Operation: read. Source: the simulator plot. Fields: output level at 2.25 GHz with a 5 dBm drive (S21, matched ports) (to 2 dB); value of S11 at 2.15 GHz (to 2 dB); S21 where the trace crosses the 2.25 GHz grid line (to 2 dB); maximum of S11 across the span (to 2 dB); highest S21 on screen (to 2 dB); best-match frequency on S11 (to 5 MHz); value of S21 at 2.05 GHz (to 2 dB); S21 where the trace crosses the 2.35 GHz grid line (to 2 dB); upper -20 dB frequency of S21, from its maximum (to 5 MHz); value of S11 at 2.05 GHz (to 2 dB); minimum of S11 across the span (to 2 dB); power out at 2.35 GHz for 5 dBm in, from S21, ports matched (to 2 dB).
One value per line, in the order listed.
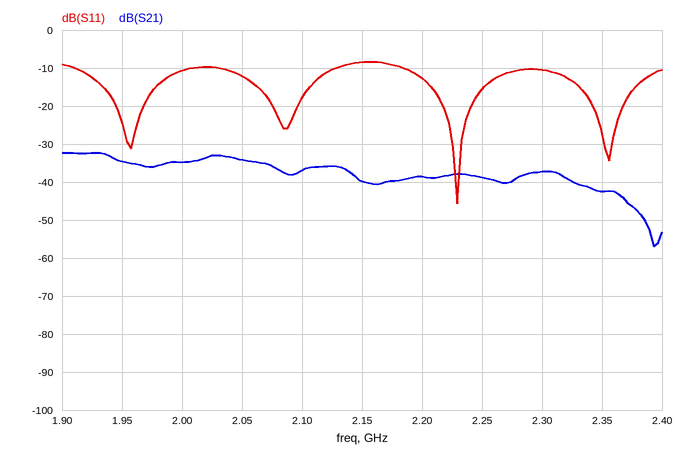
-34 dBm
-8 dB
-38 dB
-8 dB
-32 dB
2.230 GHz
-34 dB
-42 dB
2.390 GHz
-12 dB
-46 dB
-38 dBm
